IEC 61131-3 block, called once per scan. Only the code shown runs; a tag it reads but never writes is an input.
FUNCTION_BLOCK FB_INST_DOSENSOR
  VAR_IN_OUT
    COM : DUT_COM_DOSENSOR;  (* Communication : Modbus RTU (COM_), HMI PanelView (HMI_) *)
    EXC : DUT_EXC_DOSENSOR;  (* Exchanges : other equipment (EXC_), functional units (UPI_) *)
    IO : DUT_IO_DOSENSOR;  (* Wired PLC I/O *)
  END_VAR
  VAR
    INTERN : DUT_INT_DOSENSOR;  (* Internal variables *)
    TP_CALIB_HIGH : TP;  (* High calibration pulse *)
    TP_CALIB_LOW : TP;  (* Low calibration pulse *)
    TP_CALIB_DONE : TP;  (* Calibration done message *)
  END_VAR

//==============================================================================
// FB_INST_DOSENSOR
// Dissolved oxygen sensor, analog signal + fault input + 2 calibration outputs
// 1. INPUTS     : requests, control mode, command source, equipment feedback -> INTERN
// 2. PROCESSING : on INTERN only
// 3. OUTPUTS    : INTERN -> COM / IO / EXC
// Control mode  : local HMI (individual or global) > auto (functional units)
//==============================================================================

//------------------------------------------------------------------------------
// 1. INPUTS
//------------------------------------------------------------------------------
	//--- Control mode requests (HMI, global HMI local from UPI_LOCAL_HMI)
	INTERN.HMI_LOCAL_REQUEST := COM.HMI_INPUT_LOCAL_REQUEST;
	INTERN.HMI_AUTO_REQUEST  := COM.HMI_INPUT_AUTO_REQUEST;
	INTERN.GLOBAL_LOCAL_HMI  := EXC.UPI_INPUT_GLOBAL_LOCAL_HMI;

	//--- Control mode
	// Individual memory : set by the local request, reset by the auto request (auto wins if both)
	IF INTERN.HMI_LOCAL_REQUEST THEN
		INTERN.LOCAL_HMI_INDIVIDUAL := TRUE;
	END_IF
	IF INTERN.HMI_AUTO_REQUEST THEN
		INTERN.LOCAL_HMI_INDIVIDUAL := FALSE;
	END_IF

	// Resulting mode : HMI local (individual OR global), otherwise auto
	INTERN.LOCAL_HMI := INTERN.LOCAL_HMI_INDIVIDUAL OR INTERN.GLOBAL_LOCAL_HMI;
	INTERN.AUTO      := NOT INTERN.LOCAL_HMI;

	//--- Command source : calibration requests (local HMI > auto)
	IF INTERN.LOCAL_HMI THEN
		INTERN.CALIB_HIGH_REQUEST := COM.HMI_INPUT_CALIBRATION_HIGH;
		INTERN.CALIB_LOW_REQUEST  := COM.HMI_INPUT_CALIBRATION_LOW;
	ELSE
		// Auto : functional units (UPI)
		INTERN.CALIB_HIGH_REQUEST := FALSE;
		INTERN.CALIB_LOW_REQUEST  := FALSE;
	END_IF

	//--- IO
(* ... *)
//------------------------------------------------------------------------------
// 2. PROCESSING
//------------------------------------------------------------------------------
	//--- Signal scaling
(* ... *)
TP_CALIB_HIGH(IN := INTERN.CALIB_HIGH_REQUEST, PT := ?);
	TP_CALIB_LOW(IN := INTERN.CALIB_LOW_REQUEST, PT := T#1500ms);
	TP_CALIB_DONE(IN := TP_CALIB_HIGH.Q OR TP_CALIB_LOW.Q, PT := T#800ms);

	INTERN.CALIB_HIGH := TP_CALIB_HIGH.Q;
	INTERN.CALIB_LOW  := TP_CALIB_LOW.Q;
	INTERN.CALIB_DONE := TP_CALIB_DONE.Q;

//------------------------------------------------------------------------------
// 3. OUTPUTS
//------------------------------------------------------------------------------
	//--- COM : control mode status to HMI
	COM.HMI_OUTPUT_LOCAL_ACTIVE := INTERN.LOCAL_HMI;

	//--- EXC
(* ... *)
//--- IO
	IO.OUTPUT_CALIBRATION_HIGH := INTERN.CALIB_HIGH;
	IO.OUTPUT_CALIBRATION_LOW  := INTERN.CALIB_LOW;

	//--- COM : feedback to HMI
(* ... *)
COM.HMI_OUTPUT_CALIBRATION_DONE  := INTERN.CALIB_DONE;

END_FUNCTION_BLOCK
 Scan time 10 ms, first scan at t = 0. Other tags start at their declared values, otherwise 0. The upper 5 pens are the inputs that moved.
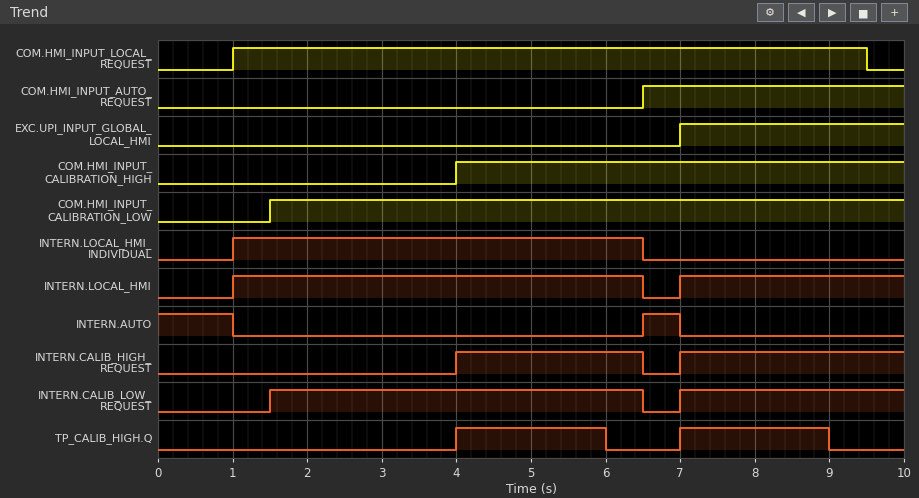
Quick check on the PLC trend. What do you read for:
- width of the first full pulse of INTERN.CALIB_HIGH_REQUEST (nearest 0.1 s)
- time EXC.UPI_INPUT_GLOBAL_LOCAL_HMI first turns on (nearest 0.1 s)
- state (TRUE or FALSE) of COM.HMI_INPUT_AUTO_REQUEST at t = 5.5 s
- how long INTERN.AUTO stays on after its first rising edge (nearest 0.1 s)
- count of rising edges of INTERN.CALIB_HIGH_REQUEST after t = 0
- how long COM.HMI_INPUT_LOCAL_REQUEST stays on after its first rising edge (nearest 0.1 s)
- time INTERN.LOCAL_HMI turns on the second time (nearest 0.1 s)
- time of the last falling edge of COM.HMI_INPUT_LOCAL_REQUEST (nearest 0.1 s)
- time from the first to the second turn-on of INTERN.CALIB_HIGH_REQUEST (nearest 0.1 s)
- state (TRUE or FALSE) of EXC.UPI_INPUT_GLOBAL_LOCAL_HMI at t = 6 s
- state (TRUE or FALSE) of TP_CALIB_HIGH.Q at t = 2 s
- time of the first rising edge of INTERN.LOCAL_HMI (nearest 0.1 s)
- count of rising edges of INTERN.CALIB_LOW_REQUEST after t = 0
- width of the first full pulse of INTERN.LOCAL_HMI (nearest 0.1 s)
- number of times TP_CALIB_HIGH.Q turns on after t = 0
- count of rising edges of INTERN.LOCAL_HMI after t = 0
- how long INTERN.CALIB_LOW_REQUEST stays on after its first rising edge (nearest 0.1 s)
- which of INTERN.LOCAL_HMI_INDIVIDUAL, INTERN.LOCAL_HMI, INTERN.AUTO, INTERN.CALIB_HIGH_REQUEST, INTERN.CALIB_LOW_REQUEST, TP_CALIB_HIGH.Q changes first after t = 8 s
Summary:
2.5 s
7.0 s
FALSE
0.5 s
2
8.5 s
7.0 s
9.5 s
3.0 s
FALSE
FALSE
1.0 s
2
5.5 s
2
2
5.0 s
TP_CALIB_HIGH.Q
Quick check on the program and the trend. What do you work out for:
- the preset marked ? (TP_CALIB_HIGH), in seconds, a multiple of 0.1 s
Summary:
2.0 s
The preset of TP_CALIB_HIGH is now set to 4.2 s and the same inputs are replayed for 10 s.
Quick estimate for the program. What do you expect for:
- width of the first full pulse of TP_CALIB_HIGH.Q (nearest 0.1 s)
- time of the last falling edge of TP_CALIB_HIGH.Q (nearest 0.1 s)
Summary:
4.2 s
8.2 s
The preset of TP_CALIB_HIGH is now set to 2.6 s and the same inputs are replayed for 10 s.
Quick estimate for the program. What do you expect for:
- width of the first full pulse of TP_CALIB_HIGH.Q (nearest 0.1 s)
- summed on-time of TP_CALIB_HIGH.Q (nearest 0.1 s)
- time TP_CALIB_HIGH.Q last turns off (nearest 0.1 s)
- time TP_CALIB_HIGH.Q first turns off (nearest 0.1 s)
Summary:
2.6 s
5.2 s
9.6 s
6.6 s
